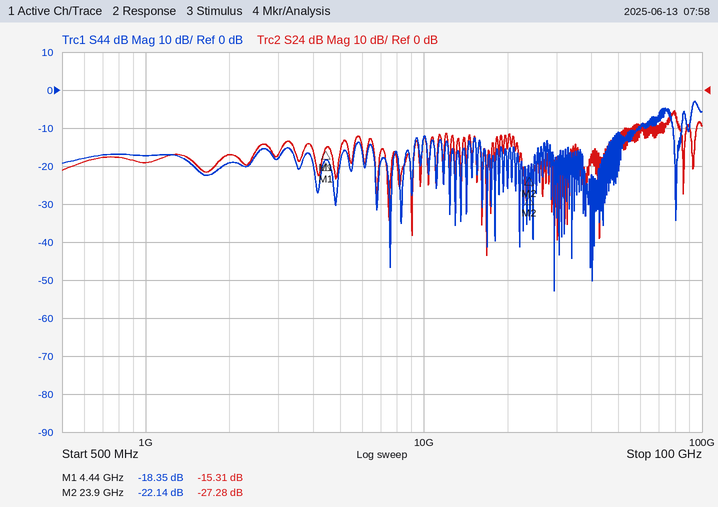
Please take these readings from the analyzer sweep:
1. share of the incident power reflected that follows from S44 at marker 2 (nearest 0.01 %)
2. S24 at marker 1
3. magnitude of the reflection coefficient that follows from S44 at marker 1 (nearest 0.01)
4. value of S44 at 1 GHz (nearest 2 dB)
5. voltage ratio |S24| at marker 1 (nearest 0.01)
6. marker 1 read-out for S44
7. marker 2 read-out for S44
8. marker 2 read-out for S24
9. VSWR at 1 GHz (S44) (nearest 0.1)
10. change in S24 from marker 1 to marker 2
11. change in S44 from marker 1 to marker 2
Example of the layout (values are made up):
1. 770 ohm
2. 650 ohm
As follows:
1. 0.61 %
2. -15.31 dB
3. 0.12
4. -18 dB
5. 0.17
6. -18.35 dB
7. -22.14 dB
8. -27.28 dB
9. 1.3
10. -11.97 dB
11. -3.79 dB
